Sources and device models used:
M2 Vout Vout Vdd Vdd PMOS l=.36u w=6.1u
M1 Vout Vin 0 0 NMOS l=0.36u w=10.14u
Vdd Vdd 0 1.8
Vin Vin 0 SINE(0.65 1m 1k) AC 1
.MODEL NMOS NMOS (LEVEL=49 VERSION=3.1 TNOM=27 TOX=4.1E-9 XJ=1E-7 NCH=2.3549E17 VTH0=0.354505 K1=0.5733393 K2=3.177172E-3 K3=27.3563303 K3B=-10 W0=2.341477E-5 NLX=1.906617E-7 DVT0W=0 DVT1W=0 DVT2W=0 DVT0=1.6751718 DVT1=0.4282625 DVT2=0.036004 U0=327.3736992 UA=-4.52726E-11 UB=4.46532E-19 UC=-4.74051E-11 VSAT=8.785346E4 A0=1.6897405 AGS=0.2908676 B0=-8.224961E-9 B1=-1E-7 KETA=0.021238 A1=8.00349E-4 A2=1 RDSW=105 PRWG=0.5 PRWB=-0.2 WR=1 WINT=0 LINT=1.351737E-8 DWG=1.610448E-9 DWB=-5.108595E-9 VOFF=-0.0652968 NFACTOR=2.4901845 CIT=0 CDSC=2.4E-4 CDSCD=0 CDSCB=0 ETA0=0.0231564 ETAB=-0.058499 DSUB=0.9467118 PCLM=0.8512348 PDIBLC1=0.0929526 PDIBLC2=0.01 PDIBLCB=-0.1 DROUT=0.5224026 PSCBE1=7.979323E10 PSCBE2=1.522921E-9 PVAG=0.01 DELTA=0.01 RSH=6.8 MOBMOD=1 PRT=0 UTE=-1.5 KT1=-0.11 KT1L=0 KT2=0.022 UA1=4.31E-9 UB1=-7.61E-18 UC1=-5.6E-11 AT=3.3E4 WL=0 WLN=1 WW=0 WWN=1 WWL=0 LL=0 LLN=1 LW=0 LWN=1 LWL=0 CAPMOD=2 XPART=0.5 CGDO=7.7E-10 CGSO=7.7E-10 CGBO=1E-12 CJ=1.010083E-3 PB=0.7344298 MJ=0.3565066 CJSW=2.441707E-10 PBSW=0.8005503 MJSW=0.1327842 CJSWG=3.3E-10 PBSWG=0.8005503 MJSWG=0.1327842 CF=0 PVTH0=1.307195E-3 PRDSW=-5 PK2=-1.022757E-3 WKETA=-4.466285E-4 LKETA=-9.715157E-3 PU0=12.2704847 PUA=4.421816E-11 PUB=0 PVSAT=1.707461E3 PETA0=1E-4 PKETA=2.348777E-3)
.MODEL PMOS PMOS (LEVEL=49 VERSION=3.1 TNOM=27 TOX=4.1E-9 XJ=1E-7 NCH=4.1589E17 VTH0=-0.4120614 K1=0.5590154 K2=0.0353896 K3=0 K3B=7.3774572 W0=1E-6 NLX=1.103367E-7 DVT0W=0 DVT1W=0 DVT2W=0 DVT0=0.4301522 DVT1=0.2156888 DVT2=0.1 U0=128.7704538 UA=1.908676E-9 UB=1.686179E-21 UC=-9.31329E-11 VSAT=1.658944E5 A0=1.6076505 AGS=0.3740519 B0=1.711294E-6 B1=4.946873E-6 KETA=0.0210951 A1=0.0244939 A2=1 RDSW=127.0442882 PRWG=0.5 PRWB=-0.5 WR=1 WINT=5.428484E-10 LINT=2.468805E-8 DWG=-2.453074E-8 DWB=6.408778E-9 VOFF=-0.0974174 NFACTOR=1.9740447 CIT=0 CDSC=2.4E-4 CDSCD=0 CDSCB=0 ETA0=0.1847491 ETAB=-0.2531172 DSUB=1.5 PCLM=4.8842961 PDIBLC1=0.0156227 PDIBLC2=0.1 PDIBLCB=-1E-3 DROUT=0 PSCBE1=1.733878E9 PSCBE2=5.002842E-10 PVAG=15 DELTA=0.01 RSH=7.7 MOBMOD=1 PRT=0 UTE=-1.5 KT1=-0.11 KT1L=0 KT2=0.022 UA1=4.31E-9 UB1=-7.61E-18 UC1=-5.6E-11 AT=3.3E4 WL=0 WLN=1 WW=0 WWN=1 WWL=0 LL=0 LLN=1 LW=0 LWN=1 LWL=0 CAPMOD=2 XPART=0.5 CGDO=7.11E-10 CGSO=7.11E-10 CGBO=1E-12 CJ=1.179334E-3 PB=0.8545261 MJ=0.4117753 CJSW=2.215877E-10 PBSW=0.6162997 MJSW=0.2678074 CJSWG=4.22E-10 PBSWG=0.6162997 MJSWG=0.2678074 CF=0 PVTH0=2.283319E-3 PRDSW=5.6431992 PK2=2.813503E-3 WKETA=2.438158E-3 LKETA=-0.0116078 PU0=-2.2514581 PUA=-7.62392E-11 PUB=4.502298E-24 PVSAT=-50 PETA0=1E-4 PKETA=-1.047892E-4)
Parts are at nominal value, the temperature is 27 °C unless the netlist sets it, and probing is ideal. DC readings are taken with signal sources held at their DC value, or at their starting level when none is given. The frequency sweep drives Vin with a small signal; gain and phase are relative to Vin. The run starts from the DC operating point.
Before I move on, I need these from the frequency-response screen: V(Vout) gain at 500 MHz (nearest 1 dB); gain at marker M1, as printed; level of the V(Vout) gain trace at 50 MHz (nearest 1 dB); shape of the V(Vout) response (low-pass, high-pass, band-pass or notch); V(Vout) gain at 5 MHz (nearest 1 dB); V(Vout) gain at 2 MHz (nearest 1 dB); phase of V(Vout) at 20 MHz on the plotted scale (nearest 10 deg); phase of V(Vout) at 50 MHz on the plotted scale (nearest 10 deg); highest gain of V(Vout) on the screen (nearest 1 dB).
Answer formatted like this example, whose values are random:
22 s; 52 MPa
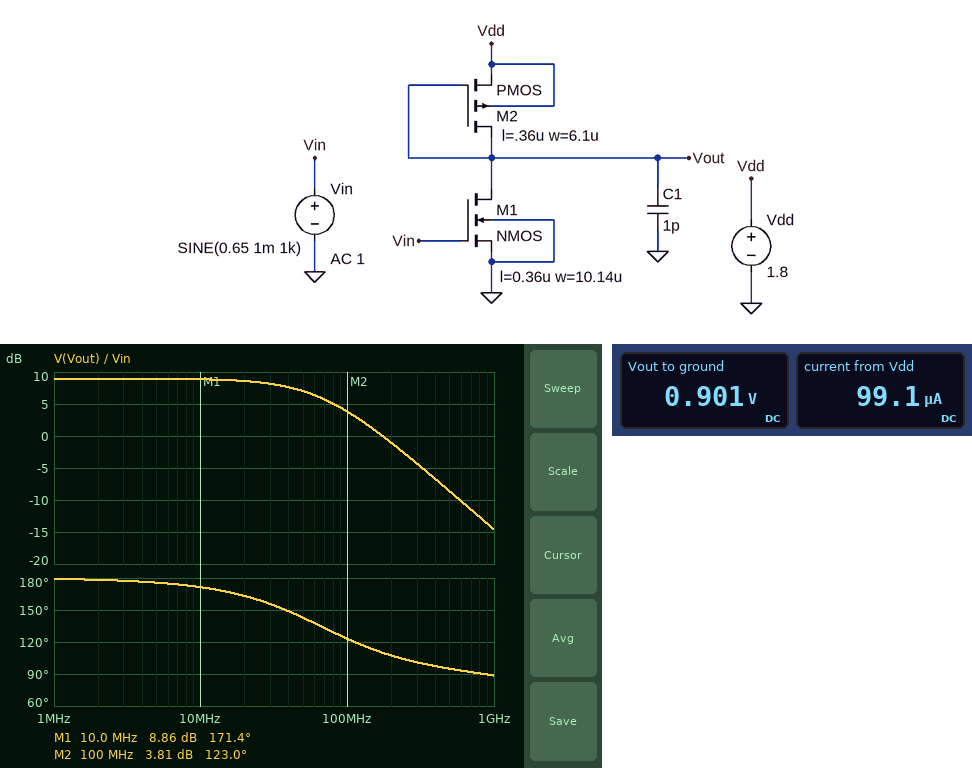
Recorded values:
-9 dB; 8.86 dB; 7 dB; low-pass; 9 dB; 9 dB; 160 deg; 140 deg; 9 dB
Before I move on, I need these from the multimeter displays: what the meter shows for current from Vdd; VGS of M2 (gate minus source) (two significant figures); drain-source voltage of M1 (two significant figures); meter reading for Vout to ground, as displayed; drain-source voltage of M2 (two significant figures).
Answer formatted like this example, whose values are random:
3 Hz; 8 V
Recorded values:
99.1 µA; -900 mV; 900 mV; 0.901 V; -900 mV
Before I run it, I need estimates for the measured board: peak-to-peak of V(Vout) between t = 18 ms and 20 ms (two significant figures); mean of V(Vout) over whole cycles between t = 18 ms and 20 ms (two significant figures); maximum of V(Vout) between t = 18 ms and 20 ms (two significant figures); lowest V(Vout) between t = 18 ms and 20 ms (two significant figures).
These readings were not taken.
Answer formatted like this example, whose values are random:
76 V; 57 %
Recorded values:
5.6 mV; 900 mV; 900 mV; 900 mV
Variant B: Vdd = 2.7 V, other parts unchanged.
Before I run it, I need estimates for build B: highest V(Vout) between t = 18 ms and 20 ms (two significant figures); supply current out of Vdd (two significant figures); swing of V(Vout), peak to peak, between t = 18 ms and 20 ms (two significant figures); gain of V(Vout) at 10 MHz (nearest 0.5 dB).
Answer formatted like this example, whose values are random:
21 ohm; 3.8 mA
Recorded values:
1.8 V; 110 µA; 5.8 mV; 9.0 dB
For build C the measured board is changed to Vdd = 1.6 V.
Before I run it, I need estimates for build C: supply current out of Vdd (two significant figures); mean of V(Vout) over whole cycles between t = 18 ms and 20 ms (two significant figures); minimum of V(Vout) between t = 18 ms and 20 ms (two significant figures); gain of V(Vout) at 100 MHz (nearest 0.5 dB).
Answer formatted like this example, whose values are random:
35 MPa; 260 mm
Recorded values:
97 µA; 710 mV; 700 mV; 3.5 dB
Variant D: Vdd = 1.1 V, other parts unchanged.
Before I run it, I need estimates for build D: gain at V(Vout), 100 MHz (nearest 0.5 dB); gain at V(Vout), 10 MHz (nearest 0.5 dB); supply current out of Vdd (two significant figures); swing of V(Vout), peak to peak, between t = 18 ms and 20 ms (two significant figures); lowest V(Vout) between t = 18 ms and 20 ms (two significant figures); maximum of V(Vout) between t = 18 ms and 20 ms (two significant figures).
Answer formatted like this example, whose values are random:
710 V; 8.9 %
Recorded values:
3.0 dB; 8.0 dB; 89 µA; 5.0 mV; 220 mV; 230 mV
